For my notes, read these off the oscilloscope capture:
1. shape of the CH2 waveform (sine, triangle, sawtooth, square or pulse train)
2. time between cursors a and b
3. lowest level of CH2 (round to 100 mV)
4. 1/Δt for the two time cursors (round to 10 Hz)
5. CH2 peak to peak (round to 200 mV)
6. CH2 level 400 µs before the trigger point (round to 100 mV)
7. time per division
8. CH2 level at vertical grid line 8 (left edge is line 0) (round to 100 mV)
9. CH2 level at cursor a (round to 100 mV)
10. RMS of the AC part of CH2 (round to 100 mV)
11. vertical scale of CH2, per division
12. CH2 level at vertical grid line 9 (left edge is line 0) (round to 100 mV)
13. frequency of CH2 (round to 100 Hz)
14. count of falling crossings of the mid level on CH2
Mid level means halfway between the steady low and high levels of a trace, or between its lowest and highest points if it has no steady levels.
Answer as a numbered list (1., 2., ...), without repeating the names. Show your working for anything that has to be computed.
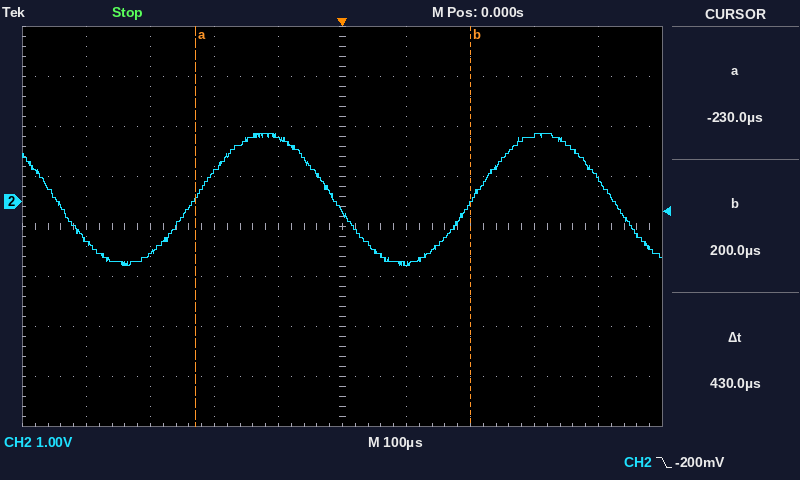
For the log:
1. sine
2. 430 µs
3. -1.3 V
4. 1 / 430 µs ≈ 2.33 kHz
5. 2.6 V
6. -800 mV
7. 100 µs
8. 1.3 V
9. 100 mV
10. 2.6 V / (2√2) ≈ 919 mV, so 900 mV to the nearest 100 mV
11. 1 V
12. 500 mV
13. 2.3 kHz
14. 3
